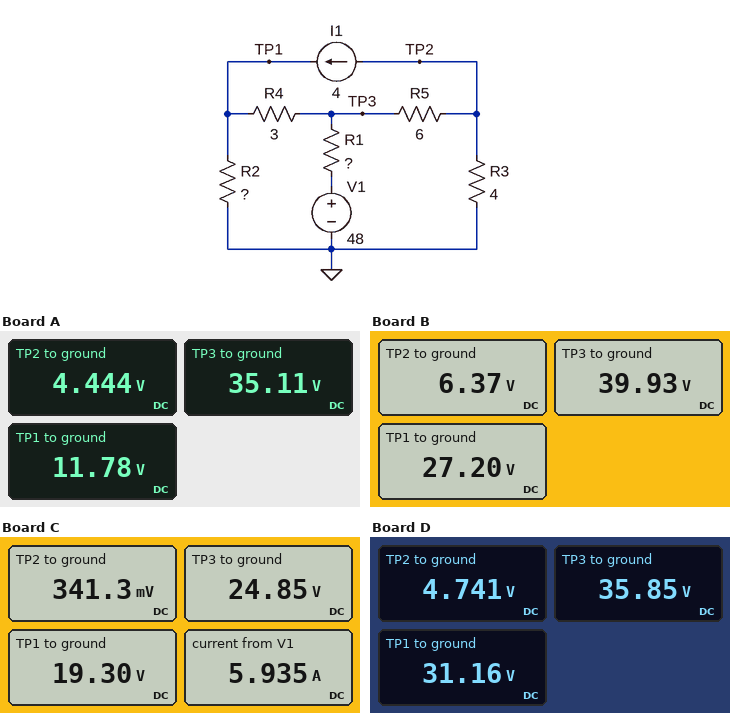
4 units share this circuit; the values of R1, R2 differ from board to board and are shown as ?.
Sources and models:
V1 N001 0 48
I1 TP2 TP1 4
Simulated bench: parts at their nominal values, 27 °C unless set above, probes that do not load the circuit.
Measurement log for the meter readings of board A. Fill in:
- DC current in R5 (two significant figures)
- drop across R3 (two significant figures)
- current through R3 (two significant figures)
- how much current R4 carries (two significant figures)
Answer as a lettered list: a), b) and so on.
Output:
a) 5.1 A
b) 4.4 V
c) 1.1 A
d) 7.8 A
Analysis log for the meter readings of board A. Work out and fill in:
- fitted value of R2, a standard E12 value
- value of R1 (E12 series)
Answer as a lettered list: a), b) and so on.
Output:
a) 1 Ω
b) 1 Ω
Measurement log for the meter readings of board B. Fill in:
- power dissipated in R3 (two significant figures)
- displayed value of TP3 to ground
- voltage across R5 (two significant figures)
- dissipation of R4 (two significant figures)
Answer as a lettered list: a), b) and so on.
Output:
a) 10 W
b) 39.93 V
c) 34 V
d) 54 W
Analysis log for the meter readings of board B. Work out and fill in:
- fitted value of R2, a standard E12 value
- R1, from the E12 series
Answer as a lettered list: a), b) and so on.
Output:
a) 3.3 Ω
b) 0.82 Ω
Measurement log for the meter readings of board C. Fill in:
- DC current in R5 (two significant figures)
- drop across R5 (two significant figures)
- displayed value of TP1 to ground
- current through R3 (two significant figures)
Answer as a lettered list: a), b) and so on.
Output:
a) 4.1 A
b) 25 V
c) 19.30 V
d) 85 mA
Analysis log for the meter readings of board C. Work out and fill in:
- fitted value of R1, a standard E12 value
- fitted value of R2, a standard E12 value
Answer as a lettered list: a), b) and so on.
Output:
a) 3.9 Ω
b) 3.3 Ω
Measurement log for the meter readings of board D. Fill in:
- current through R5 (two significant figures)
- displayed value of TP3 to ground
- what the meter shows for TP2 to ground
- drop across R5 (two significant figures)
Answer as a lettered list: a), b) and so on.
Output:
a) 5.2 A
b) 35.85 V
c) 4.741 V
d) 31 V
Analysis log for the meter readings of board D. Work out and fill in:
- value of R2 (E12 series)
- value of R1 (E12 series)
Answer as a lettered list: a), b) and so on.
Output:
a) 5.6 Ω
b) 1.8 Ω
